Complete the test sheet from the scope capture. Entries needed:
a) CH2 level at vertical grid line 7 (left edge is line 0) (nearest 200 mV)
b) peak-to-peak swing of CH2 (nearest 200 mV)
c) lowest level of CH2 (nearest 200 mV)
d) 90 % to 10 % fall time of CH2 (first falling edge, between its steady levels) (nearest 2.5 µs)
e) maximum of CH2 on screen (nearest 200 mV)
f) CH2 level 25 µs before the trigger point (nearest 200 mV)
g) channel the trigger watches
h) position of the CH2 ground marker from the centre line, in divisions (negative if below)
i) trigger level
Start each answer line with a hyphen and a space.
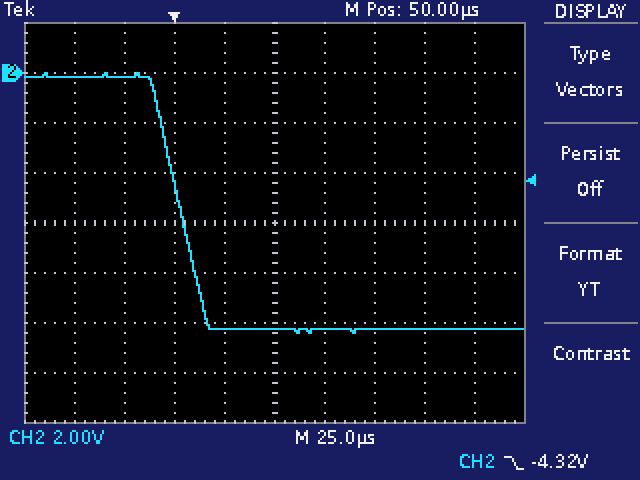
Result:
- -10.2 V
- 10.4 V
- -10.4 V
- 22.5 µs
- 0.0 V
- -200 mV
- CH2
- +3.0 div
- -4.32 V
